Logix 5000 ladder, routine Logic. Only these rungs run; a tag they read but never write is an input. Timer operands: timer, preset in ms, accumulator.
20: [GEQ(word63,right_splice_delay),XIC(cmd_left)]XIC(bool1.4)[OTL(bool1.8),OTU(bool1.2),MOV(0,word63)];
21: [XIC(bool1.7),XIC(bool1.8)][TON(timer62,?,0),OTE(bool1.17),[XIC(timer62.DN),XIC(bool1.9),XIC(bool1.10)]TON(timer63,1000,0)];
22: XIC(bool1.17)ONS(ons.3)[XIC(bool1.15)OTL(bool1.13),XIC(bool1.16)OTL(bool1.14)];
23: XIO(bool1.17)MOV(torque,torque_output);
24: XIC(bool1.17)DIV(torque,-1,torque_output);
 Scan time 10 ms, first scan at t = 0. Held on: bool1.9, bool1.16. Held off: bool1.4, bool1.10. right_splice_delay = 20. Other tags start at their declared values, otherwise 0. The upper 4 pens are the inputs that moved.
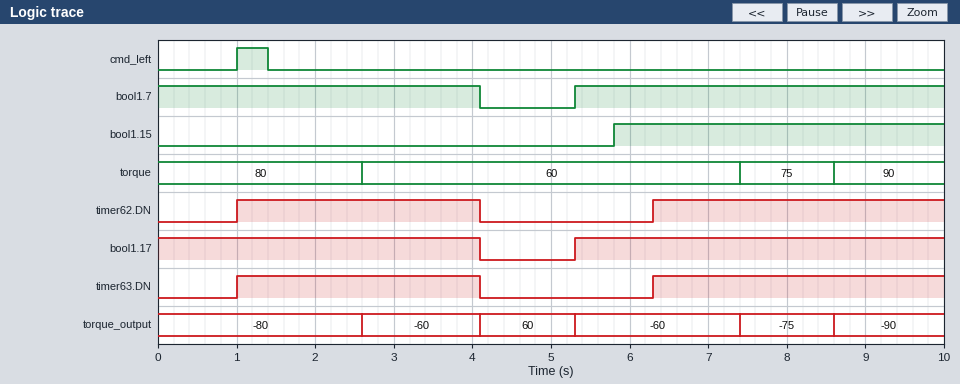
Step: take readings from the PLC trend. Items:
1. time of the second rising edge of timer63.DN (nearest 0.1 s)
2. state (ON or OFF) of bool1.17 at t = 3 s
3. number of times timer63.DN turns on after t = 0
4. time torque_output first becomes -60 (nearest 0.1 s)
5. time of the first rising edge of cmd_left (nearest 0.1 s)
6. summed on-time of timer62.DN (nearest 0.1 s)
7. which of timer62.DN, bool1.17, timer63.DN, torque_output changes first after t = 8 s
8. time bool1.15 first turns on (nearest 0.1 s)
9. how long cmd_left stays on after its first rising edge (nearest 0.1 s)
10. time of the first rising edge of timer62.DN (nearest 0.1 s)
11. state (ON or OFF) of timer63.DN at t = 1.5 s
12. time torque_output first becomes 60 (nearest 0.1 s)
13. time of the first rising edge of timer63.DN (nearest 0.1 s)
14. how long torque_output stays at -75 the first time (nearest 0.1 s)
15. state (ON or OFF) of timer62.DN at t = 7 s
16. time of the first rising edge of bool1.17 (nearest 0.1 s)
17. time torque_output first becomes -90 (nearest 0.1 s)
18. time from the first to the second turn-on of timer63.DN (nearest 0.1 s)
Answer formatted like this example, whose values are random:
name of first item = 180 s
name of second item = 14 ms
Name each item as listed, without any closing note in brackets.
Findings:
time of the second rising edge of timer63.DN = 6.3 s
state (ON or OFF) of bool1.17 at t = 3 s = ON
number of times timer63.DN turns on after t = 0 = 2
time torque_output first becomes -60 = 2.6 s
time of the first rising edge of cmd_left = 1.0 s
summed on-time of timer62.DN = 6.8 s
which of timer62.DN, bool1.17, timer63.DN, torque_output changes first after t = 8 s = torque_output
time bool1.15 first turns on = 5.8 s
how long cmd_left stays on after its first rising edge = 0.4 s
time of the first rising edge of timer62.DN = 1.0 s
state (ON or OFF) of timer63.DN at t = 1.5 s = ON
time torque_output first becomes 60 = 4.1 s
time of the first rising edge of timer63.DN = 1.0 s
how long torque_output stays at -75 the first time = 1.2 s
state (ON or OFF) of timer62.DN at t = 7 s = ON
time of the first rising edge of bool1.17 = 5.3 s
time torque_output first becomes -90 = 8.6 s
time from the first to the second turn-on of timer63.DN = 5.3 s
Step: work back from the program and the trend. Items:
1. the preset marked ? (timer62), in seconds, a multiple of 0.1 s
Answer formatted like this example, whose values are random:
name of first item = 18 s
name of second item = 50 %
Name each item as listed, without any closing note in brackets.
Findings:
the preset marked ? (timer62), in seconds, a multiple of 0.1 s = 1.0 s
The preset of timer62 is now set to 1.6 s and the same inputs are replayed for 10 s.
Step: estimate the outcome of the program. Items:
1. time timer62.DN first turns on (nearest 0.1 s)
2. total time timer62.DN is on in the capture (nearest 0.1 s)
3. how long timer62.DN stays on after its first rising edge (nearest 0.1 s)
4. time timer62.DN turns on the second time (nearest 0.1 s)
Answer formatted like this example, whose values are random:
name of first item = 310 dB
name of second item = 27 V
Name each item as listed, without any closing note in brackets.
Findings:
time timer62.DN first turns on = 1.6 s
total time timer62.DN is on in the capture = 5.6 s
how long timer62.DN stays on after its first rising edge = 2.5 s
time timer62.DN turns on the second time = 6.9 s
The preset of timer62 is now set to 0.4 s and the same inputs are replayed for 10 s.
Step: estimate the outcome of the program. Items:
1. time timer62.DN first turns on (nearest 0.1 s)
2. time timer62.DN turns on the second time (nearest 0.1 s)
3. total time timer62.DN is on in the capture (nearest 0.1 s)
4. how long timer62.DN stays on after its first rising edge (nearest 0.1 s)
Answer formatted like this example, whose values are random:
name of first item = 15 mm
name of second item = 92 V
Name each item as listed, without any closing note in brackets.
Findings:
time timer62.DN first turns on = 0.4 s
time timer62.DN turns on the second time = 5.7 s
total time timer62.DN is on in the capture = 8.0 s
how long timer62.DN stays on after its first rising edge = 3.7 s
